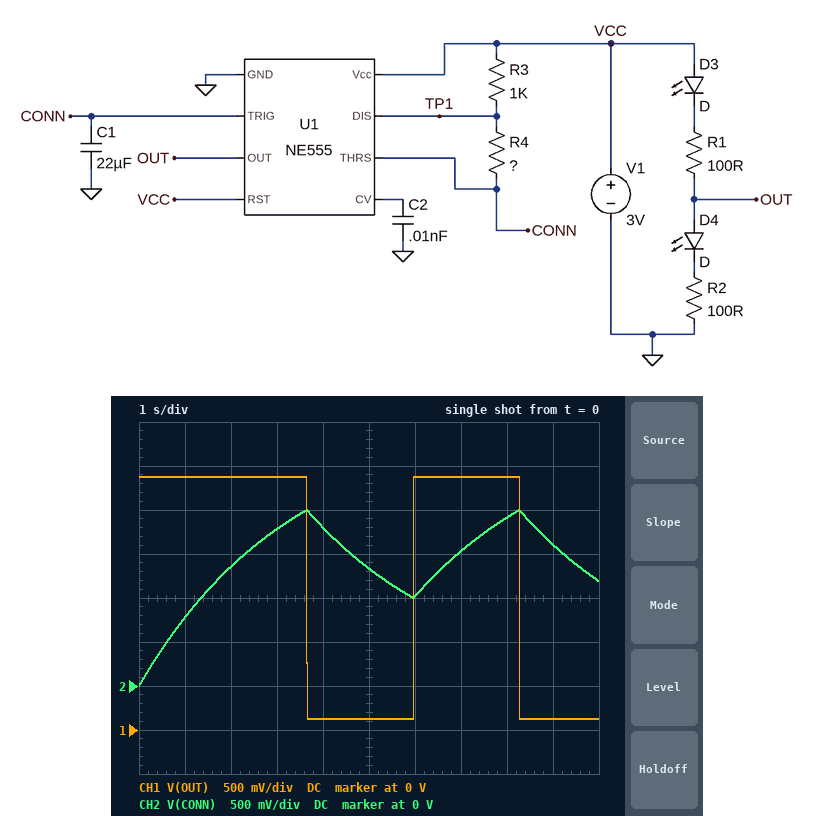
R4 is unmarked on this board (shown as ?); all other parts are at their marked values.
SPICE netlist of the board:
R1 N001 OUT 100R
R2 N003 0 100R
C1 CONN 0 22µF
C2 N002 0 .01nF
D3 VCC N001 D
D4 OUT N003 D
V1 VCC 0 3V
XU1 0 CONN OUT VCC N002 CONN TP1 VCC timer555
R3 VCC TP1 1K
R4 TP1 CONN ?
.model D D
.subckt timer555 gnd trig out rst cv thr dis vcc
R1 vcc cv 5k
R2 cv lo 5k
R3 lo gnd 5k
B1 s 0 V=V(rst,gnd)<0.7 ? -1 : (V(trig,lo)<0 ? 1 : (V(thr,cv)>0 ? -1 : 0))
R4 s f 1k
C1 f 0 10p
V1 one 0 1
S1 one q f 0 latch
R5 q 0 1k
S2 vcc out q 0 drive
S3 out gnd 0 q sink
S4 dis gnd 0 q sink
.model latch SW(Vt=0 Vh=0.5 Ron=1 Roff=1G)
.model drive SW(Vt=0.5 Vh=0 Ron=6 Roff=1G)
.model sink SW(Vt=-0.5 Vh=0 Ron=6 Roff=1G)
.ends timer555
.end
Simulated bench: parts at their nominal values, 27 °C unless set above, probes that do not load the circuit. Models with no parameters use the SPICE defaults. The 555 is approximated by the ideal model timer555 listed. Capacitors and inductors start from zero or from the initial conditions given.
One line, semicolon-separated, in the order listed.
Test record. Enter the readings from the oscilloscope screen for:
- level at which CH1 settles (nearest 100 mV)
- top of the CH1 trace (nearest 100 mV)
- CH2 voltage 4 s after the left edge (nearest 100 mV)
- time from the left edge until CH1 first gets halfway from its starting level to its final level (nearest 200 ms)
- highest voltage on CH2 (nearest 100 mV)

100 mV; 2.9 V; 1.8 V; 3.6 s; 2.0 V
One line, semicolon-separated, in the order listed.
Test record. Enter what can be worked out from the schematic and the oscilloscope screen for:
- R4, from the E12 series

150 kΩ
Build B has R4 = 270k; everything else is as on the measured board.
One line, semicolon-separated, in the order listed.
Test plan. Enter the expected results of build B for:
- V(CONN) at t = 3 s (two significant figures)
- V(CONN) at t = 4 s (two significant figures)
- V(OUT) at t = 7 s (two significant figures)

1.2 V; 1.5 V; 130 mV
